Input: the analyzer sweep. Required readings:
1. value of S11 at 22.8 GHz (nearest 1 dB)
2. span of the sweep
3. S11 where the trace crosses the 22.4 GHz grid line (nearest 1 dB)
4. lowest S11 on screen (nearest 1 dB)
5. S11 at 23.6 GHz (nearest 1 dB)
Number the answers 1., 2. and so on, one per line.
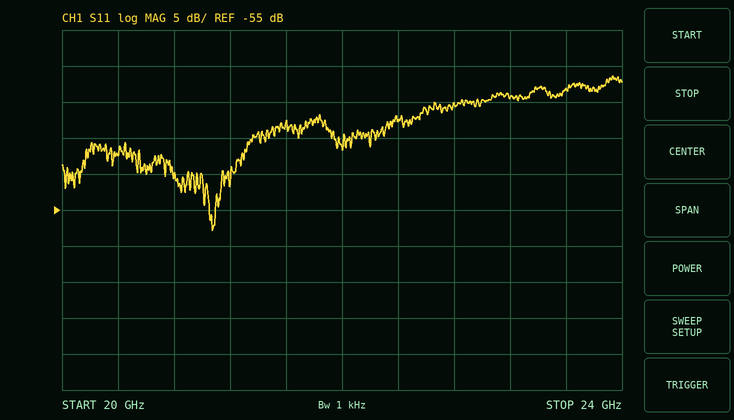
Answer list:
1. -40 dB
2. 4 GHz
3. -43 dB
4. -58 dB
5. -38 dB
